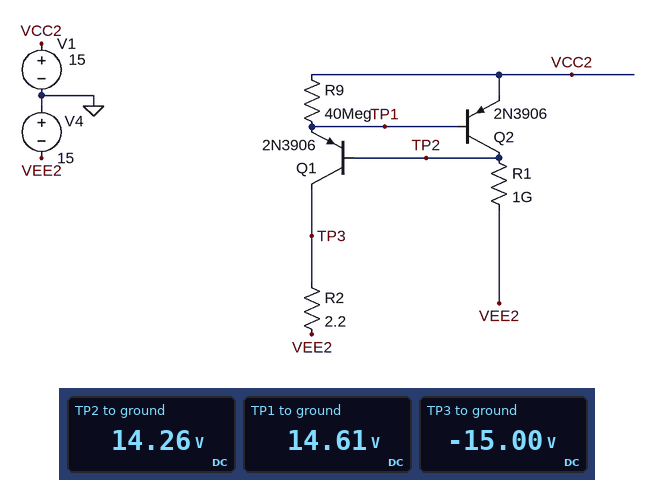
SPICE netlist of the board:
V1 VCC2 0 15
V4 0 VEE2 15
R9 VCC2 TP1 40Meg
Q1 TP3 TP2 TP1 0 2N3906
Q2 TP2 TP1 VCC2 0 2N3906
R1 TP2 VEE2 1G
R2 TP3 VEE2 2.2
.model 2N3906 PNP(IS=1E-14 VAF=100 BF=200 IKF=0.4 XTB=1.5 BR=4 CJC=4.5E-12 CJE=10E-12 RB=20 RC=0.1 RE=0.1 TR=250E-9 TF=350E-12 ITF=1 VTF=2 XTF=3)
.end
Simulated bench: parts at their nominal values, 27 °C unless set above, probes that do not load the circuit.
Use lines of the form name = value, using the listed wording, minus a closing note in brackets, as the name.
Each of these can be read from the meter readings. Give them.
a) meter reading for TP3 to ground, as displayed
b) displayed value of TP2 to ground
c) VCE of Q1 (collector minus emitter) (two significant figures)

meter reading for TP3 to ground, as displayed = -15.00 V
displayed value of TP2 to ground = 14.26 V
VCE of Q1 (collector minus emitter) = -30 V
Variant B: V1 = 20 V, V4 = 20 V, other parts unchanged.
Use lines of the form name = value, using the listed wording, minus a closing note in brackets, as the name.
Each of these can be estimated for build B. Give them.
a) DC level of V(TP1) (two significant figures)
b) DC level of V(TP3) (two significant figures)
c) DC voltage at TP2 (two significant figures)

DC level of V(TP1) = 20 V
DC level of V(TP3) = -20 V
DC voltage at TP2 = 19 V
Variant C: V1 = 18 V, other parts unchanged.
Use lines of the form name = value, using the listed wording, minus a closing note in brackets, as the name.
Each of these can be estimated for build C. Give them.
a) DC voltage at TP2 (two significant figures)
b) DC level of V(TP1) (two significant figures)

DC voltage at TP2 = 17 V
DC level of V(TP1) = 18 V
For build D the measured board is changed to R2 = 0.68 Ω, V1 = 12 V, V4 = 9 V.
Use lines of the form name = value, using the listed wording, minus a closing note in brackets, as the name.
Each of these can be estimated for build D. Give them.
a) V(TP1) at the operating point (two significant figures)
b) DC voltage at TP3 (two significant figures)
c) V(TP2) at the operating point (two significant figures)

V(TP1) at the operating point = 12 V
DC voltage at TP3 = -9.0 V
V(TP2) at the operating point = 11 V
